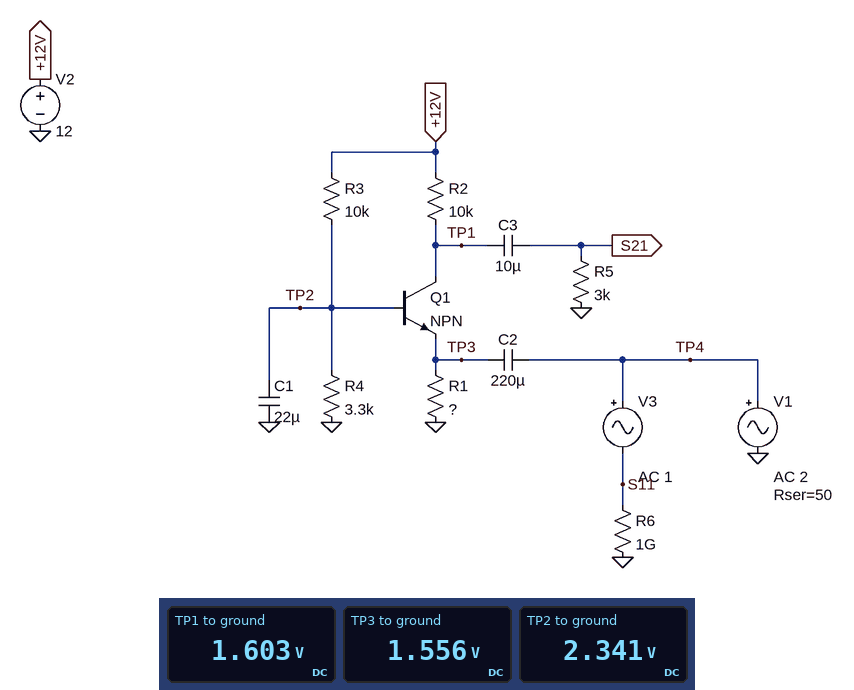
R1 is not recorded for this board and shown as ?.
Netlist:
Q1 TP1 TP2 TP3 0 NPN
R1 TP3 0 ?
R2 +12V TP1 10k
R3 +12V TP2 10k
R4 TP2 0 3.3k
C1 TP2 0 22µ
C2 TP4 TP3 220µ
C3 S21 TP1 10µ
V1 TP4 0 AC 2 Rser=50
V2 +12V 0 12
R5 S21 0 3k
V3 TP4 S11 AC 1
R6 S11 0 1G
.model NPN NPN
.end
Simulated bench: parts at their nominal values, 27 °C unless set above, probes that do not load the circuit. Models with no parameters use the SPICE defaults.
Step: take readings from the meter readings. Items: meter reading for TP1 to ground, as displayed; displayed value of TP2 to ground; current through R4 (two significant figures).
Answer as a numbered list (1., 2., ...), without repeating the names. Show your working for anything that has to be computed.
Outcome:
1. 1.603 V
2. 2.341 V
3. (2.341 V) / 3.3 kΩ = 710 µA
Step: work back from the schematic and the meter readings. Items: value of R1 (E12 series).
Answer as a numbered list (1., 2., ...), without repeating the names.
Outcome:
1. 1.2 kΩ
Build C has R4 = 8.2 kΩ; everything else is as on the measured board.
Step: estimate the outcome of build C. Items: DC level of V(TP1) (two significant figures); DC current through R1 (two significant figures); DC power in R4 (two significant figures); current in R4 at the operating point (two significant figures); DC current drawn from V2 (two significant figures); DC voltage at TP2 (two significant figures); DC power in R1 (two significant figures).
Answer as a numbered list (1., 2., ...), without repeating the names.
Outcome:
1. 2.0 V
2. 1.6 mA
3. 900 µW
4. 330 µA
5. 1.9 mA
6. 2.7 V
7. 3.1 mW
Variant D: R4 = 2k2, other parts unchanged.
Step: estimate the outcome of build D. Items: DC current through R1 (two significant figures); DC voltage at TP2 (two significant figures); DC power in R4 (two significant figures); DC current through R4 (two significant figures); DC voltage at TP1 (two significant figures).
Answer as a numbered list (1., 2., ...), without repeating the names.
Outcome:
1. 1.1 mA
2. 2.1 V
3. 2.0 mW
4. 950 µA
5. 1.4 V
